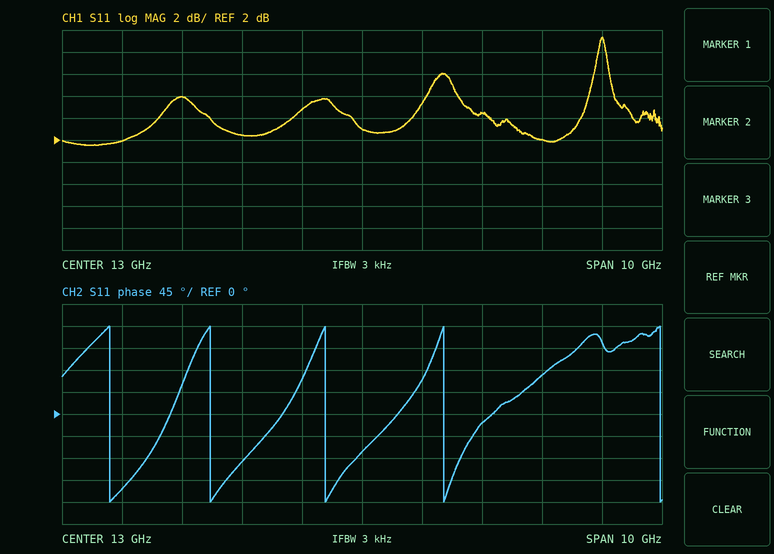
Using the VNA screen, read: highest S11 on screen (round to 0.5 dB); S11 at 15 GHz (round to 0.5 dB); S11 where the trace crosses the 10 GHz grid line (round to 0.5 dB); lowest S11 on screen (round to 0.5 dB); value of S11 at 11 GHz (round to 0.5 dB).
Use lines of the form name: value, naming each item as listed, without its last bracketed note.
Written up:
highest S11 on screen: 11.5 dB
S11 at 15 GHz: 4.5 dB
S11 where the trace crosses the 10 GHz grid line: 6.0 dB
lowest S11 on screen: 1.5 dB
value of S11 at 11 GHz: 2.5 dB
